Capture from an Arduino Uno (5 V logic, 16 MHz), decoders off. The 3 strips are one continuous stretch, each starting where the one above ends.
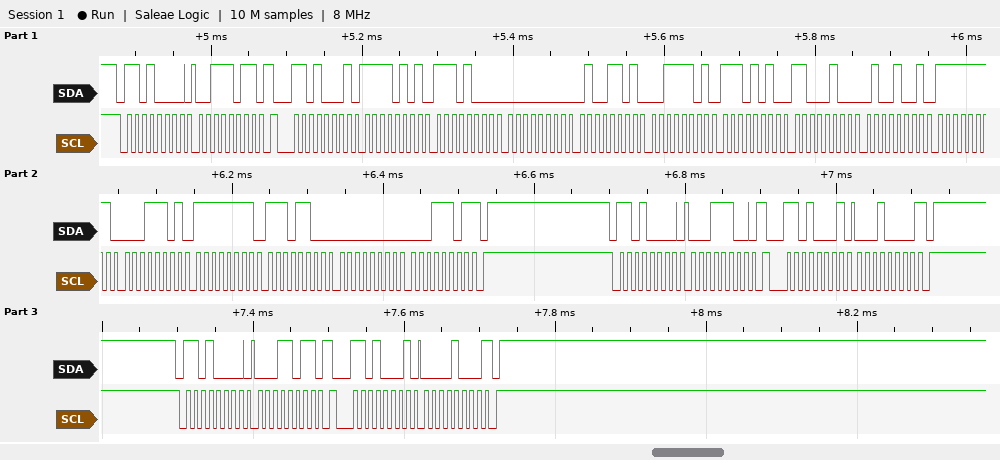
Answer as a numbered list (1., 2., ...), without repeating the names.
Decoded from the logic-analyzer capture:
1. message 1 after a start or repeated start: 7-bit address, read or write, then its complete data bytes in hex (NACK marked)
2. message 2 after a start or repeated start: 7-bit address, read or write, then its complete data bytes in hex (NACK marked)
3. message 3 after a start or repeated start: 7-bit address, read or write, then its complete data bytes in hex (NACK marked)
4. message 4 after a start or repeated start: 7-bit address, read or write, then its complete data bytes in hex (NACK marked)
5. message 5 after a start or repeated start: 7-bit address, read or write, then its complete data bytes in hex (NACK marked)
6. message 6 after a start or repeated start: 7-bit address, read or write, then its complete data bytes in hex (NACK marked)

1. 0x68 write: 3B
2. 0x68 read: F5 E8 00 4D 3D EA C4 49 FF 1D FF EC 00 1D NACK
3. 0x68 write: 1C
4. 0x68 read: 10 NACK
5. 0x68 write: 1B
6. 0x68 read: 08 NACK
